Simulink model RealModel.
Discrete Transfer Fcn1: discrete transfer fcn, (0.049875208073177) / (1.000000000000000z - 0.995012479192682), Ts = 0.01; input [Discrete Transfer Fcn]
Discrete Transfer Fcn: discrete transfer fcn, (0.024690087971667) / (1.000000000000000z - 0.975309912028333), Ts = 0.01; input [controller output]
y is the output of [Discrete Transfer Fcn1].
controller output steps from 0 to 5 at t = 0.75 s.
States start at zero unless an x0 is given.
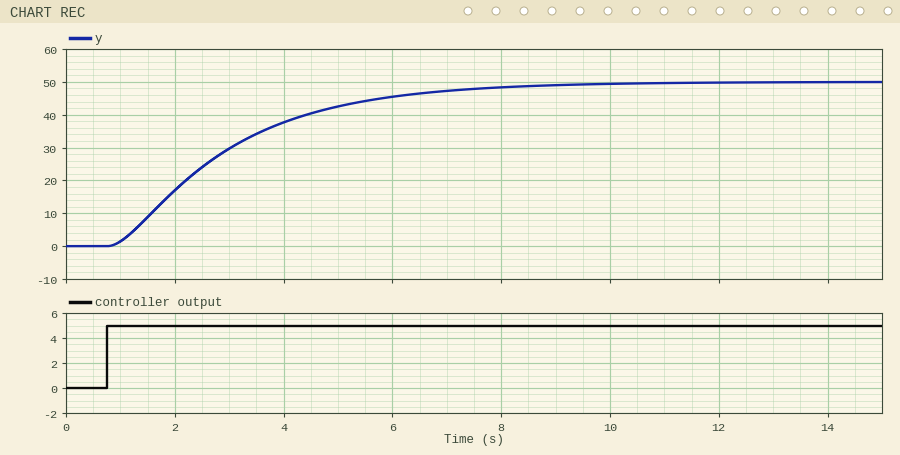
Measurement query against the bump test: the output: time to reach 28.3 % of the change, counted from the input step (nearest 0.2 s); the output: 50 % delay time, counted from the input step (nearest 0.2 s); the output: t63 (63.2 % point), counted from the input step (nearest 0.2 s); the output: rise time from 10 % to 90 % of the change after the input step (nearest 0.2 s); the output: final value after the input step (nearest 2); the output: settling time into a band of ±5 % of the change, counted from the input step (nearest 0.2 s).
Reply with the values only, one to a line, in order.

1.0 s
1.8 s
2.4 s
4.6 s
50
6.4 s
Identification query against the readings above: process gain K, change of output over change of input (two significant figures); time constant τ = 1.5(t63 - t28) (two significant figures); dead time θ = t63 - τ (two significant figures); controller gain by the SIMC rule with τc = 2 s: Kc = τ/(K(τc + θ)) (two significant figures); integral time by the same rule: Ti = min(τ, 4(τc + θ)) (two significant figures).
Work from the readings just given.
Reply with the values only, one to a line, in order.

10
2.1 s
0.30 s
0.091
2.1 s
